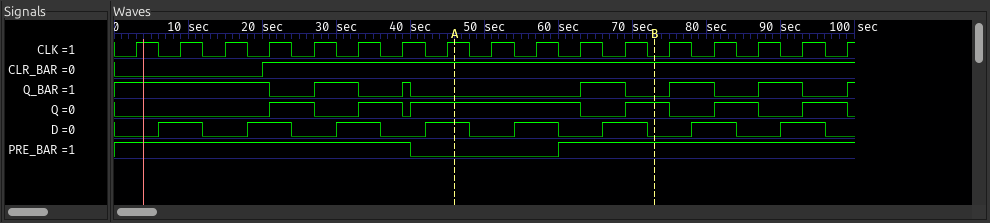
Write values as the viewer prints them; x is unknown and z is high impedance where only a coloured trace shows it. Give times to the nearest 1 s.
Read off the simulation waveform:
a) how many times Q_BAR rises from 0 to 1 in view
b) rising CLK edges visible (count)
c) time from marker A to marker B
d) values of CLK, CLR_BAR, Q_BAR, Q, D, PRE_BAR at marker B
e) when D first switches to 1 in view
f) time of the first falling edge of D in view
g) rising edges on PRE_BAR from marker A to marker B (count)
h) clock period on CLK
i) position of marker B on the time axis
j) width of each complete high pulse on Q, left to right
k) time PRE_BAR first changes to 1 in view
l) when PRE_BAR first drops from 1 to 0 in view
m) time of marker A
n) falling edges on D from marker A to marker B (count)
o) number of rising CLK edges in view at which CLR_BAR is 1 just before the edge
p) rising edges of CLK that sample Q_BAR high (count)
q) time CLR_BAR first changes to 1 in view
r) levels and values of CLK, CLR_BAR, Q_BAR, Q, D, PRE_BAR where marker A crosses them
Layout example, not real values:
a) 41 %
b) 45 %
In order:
a) 6
b) 17
c) 27 s
d) CLK=0, CLR_BAR=1, Q_BAR=0, Q=1, D=0, PRE_BAR=1
e) 6 s
f) 12 s
g) 1
h) 6 s
i) 73 s
j) 6 s, 6 s, 23 s, 6 s, 6 s, 6 s
k) 60 s
l) 40 s
m) 46 s
n) 3
o) 14
p) 8
q) 20 s
r) CLK=1, CLR_BAR=1, Q_BAR=0, Q=1, D=1, PRE_BAR=0
